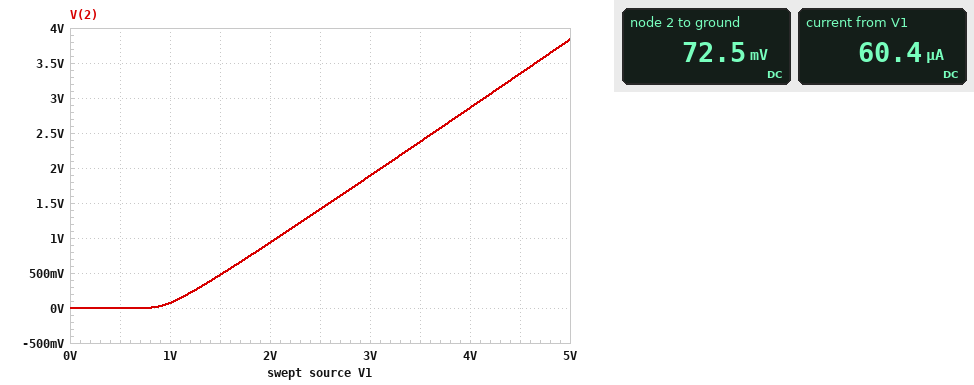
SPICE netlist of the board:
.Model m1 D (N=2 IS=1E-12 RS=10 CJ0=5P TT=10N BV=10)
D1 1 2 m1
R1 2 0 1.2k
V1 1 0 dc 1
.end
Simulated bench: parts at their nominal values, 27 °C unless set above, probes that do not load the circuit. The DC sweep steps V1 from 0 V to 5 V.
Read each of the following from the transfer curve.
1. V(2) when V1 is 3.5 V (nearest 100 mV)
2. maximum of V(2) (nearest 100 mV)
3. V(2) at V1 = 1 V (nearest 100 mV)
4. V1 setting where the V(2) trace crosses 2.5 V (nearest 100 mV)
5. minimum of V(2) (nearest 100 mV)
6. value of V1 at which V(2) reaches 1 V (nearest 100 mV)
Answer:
2.4 V
3.8 V
100 mV
3.6 V
0 V
2.1 V
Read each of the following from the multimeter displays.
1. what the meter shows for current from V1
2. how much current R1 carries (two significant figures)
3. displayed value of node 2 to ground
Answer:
60.4 µA
60 µA
72.5 mV
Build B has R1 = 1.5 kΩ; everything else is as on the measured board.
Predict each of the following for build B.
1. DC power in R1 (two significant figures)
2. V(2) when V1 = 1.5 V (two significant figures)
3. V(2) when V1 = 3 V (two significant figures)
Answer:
4.2 µW
480 mV
1.9 V
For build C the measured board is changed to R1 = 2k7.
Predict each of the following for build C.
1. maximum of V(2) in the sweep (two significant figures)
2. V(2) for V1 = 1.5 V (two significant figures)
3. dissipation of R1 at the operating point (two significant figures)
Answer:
3.9 V
510 mV
3.6 µW
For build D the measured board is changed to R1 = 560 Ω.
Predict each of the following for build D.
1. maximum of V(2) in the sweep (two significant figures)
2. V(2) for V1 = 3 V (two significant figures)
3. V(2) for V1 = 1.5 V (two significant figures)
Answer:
3.8 V
1.8 V
430 mV
